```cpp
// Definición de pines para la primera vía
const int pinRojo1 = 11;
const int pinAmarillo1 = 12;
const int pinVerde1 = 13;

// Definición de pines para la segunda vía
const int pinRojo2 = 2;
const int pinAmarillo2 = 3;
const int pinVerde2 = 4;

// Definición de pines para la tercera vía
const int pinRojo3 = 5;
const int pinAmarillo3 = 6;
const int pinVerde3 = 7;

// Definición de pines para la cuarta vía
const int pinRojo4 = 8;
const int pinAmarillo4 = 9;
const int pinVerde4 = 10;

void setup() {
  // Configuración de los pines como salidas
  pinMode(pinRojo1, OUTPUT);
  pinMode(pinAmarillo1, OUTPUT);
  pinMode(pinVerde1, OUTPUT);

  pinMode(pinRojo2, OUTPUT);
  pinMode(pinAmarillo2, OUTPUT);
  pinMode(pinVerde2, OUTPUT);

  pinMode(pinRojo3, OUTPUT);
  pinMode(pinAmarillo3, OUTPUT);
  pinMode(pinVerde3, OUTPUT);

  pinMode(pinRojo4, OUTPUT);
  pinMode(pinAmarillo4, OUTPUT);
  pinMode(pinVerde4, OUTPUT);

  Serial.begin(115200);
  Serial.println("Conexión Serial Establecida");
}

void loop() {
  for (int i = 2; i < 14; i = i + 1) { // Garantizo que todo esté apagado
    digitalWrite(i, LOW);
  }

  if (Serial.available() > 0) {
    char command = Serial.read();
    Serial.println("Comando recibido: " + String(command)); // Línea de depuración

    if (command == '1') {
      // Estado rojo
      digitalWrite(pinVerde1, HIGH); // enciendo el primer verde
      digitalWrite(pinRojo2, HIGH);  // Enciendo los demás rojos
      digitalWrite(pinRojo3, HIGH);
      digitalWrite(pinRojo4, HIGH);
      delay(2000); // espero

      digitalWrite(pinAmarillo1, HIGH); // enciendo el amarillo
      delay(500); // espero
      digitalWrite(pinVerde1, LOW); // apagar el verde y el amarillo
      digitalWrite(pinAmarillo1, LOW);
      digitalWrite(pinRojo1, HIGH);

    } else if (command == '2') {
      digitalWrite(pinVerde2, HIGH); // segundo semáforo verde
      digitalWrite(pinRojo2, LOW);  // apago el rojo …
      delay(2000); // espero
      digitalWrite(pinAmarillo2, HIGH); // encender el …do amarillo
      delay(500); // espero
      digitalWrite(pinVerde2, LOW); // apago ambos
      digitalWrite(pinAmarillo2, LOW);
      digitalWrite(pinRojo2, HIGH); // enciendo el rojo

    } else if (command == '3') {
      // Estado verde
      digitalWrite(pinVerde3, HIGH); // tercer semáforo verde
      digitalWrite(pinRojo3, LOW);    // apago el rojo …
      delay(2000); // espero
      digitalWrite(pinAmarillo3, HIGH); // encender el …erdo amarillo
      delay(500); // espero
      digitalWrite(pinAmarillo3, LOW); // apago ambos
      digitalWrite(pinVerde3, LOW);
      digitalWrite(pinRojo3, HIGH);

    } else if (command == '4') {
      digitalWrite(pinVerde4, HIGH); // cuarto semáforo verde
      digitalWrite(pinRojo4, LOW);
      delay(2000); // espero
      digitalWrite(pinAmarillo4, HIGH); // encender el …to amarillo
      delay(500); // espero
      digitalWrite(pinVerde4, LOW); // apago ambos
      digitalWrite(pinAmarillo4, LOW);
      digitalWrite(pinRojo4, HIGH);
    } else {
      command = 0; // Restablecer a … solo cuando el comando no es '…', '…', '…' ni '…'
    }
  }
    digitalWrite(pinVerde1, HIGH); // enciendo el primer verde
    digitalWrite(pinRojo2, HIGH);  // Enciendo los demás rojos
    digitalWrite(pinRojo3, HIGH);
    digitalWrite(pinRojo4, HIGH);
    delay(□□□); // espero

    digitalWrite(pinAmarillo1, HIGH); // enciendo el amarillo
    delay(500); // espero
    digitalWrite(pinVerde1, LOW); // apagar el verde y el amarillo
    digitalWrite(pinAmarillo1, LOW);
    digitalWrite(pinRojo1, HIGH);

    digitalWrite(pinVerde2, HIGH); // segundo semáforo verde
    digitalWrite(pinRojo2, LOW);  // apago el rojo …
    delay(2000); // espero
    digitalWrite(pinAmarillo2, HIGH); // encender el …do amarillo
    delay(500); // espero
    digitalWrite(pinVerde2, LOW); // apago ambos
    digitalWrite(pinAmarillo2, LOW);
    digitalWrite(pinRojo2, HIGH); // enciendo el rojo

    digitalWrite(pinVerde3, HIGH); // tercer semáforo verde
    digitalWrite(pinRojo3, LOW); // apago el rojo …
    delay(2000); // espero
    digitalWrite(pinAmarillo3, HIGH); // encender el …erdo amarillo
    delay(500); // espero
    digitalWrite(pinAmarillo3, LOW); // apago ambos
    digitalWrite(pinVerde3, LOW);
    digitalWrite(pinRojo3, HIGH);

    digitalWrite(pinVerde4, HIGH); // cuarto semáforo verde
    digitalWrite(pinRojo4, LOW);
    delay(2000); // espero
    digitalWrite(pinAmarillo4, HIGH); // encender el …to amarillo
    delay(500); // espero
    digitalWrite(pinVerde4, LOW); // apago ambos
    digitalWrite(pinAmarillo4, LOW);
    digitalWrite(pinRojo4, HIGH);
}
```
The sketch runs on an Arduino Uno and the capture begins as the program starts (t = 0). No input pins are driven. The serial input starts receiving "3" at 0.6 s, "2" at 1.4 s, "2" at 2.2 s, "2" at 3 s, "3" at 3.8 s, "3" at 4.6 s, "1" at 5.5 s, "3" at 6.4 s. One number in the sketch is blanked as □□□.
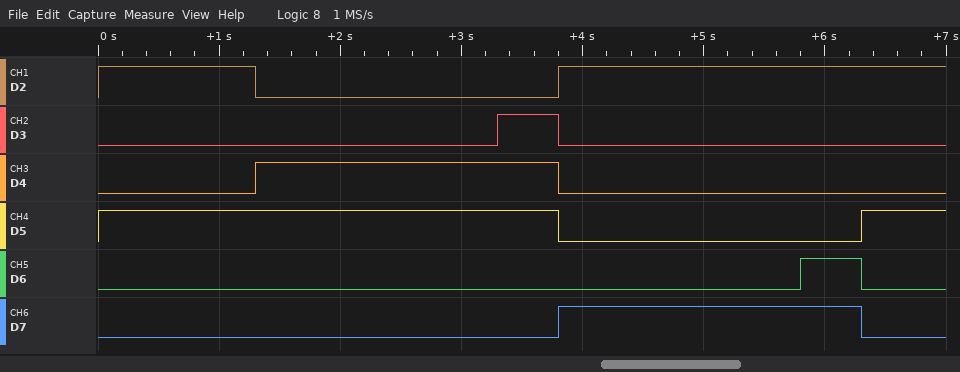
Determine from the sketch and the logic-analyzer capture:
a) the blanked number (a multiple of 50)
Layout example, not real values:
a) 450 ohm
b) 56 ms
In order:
a) 800
